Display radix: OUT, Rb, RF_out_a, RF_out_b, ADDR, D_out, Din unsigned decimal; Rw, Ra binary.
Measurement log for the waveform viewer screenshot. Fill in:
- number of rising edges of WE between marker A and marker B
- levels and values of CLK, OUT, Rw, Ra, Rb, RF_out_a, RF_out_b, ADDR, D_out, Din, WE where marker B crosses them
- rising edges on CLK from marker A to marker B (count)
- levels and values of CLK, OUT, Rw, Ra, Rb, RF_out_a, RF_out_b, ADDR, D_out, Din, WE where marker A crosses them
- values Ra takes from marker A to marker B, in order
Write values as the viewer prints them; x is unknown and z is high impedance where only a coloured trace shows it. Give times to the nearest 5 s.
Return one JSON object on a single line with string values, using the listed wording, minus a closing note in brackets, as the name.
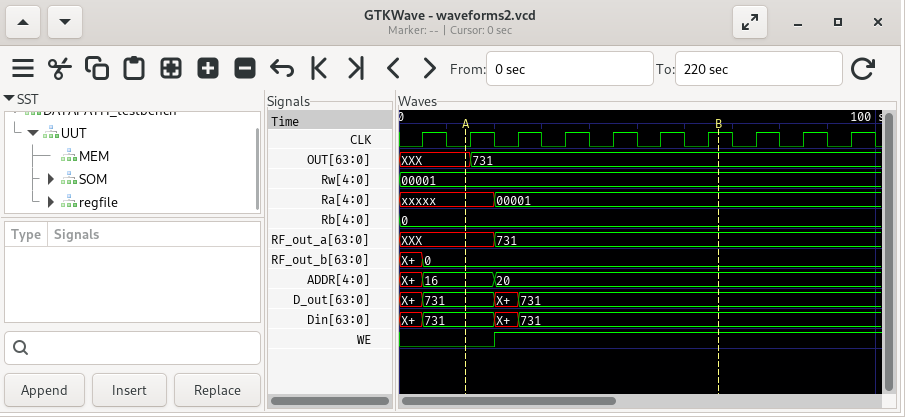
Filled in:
{"number of rising edges of WE between marker A and marker B": "1", "levels and values of CLK, OUT, Rw, Ra, Rb, RF_out_a, RF_out_b, ADDR, D_out, Din, WE where marker B crosses them": "CLK=1, OUT=731, Rw=00001, Ra=00001, Rb=0, RF_out_a=731, RF_out_b=0, ADDR=20, D_out=731, Din=731, WE=1", "rising edges on CLK from marker A to marker B": "6", "levels and values of CLK, OUT, Rw, Ra, Rb, RF_out_a, RF_out_b, ADDR, D_out, Din, WE where marker A crosses them": "CLK=0, OUT=XXX, Rw=00001, Ra=xxxxx, Rb=0, RF_out_a=XXX, RF_out_b=0, ADDR=16, D_out=731, Din=731, WE=0", "values Ra takes from marker A to marker B, in order": "xxxxx, 00001"}
